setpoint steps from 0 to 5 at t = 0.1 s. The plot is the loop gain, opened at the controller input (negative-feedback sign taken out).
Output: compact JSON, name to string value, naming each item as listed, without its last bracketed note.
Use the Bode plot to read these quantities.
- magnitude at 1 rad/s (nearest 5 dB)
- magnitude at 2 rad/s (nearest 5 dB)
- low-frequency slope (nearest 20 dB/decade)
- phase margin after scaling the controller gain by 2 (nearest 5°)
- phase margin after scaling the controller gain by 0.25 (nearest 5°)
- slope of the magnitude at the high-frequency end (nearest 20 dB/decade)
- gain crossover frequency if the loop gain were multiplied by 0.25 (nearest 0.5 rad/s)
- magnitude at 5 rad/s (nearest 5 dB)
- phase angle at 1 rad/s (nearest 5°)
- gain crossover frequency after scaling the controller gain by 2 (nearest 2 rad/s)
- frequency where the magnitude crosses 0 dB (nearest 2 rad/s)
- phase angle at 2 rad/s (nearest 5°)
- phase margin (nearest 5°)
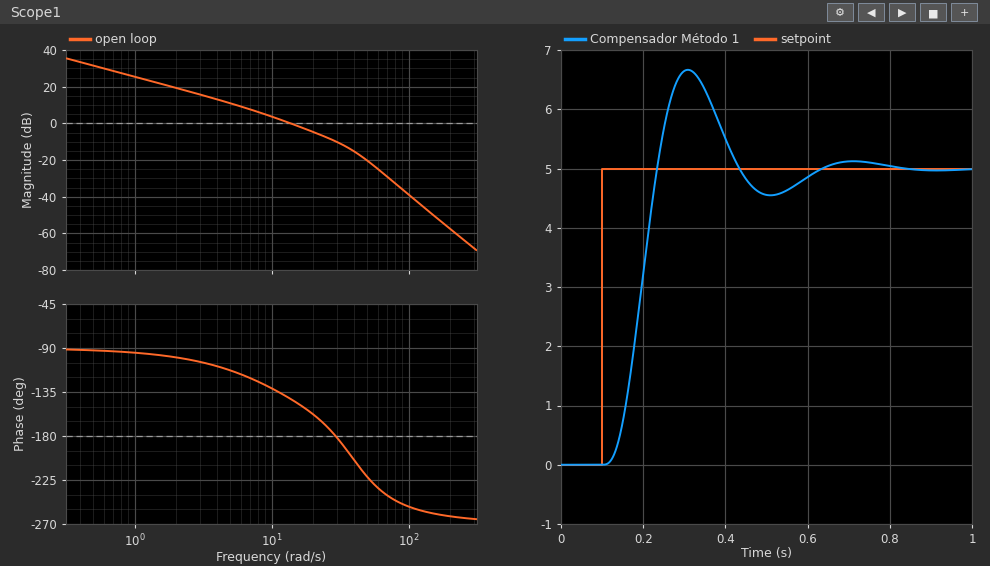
{"magnitude at 1 rad/s": "25 dB", "magnitude at 2 rad/s": "20 dB", "low-frequency slope": "-20 dB/decade", "phase margin after scaling the controller gain by 2": "15°", "phase margin after scaling the controller gain by 0.25": "70°", "slope of the magnitude at the high-frequency end": "-60 dB/decade", "gain crossover frequency if the loop gain were multiplied by 0.25": "4.5 rad/s", "magnitude at 5 rad/s": "10 dB", "phase angle at 1 rad/s": "-95°", "gain crossover frequency after scaling the controller gain by 2": "22 rad/s", "frequency where the magnitude crosses 0 dB": "14 rad/s", "phase angle at 2 rad/s": "-100°", "phase margin": "40°"}
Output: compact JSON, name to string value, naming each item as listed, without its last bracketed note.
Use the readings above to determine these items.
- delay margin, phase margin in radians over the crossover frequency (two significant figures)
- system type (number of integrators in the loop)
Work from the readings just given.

{"delay margin, phase margin in radians over the crossover frequency": "0.050 s", "system type": "1"}
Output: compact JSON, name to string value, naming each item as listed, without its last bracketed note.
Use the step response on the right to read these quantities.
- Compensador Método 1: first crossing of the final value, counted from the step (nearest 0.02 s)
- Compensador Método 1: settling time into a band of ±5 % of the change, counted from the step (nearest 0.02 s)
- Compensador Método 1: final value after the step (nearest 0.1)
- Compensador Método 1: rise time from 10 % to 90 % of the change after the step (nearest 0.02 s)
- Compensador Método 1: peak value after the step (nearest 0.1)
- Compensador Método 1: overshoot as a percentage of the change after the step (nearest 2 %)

{"Compensador Método 1: first crossing of the final value, counted from the step": "0.14 s", "Compensador Método 1: settling time into a band of ±5 % of the change, counted from the step": "0.48 s", "Compensador Método 1: final value after the step": "5.0", "Compensador Método 1: rise time from 10 % to 90 % of the change after the step": "0.08 s", "Compensador Método 1: peak value after the step": "6.7", "Compensador Método 1: overshoot as a percentage of the change after the step": "34 %"}
